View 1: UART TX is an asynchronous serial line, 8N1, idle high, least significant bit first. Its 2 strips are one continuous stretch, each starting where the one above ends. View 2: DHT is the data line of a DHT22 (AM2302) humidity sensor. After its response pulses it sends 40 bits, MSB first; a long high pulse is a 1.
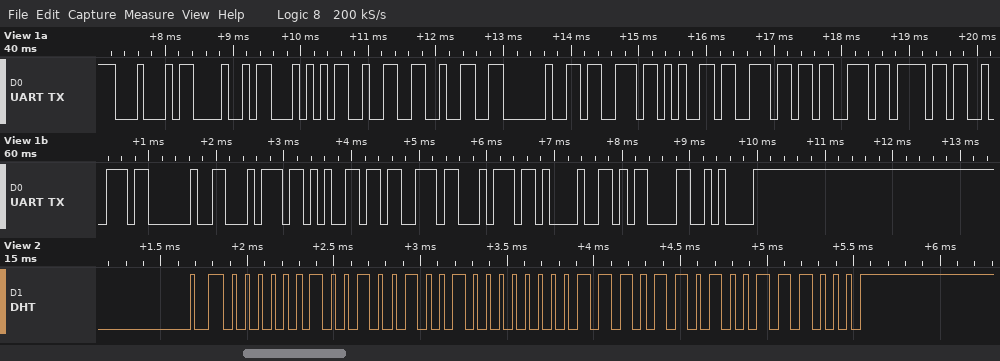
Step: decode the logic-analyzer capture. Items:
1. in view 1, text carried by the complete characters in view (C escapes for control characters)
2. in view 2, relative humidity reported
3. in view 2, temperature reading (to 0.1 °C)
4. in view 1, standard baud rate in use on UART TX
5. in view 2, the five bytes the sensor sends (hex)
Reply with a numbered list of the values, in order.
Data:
1. "DHT22 sensor test!\r\n"
2. 58.5 %
3. 23.7 °C
4. 9600 baud
5. 02 49 00 ED 38
